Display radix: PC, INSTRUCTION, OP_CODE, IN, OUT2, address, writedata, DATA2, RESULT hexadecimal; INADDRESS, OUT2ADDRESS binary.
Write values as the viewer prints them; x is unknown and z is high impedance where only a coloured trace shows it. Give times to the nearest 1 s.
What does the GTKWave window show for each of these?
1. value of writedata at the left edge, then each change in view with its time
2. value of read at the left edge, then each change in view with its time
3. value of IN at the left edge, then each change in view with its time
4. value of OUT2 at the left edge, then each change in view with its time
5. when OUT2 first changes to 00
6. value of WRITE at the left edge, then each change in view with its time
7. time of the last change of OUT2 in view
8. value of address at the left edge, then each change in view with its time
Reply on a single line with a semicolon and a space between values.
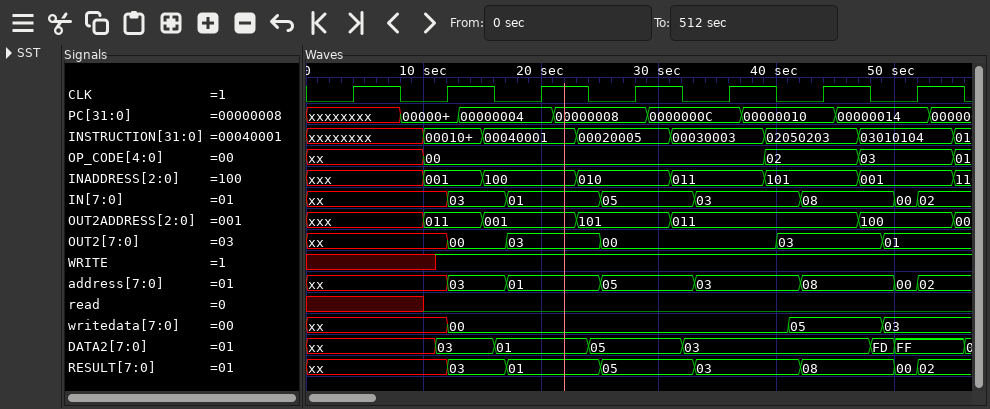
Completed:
xx, 00 at 12 s, 05 at 41 s, 03 at 49 s; x, 0 at 10 s; xx, 03 at 12 s, 01 at 17 s, 05 at 25 s, 03 at 33 s, 08 at 42 s, 00 at 50 s, 02 at 52 s; xx, 00 at 12 s, 03 at 17 s, 00 at 25 s, 03 at 40 s, 01 at 49 s; 12 s; x, 1 at 11 s; 49 s; xx, 03 at 12 s, 01 at 17 s, 05 at 25 s, 03 at 33 s, 08 at 42 s, 00 at 50 s, 02 at 52 s
